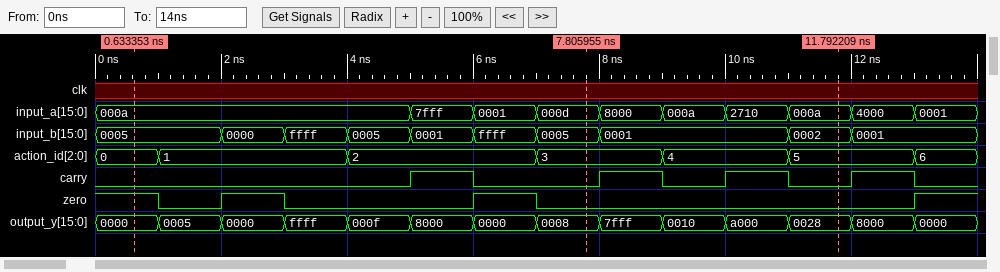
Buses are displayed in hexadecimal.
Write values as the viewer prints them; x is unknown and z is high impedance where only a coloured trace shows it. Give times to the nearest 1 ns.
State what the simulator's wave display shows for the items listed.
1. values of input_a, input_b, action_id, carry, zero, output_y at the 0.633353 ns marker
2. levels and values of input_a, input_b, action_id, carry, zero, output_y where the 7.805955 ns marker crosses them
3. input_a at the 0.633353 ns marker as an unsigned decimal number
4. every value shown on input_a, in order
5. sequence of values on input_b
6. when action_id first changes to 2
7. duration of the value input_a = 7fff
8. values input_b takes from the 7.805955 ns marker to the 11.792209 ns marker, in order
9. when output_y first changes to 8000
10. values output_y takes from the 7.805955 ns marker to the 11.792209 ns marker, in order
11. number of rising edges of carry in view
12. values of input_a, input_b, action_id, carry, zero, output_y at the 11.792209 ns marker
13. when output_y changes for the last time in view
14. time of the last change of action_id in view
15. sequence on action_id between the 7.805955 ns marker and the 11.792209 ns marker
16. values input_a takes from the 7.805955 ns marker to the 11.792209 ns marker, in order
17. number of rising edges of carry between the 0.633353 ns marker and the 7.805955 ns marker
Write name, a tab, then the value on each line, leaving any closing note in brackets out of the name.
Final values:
values of input_a, input_b, action_id, carry, zero, output_y at the 0.633353 ns marker	input_a=000a, input_b=0005, action_id=0, carry=0, zero=1, output_y=0000
levels and values of input_a, input_b, action_id, carry, zero, output_y where the 7.805955 ns marker crosses them	input_a=000d, input_b=0005, action_id=3, carry=0, zero=0, output_y=0008
input_a at the 0.633353 ns marker as an unsigned decimal number	10
every value shown on input_a, in order	000a, 7fff, 0001, 000d, 8000, 000a, 2710, 000a, 4000, 0001
sequence of values on input_b	0005, 0000, ffff, 0005, 0001, ffff, 0005, 0001, 0002, 0001
when action_id first changes to 2	4 ns
duration of the value input_a = 7fff	1 ns
values input_b takes from the 7.805955 ns marker to the 11.792209 ns marker, in order	0005, 0001, 0002
when output_y first changes to 8000	5 ns
values output_y takes from the 7.805955 ns marker to the 11.792209 ns marker, in order	0008, 7fff, 0010, a000, 0028
number of rising edges of carry in view	4
values of input_a, input_b, action_id, carry, zero, output_y at the 11.792209 ns marker	input_a=000a, input_b=0002, action_id=5, carry=0, zero=0, output_y=0028
when output_y changes for the last time in view	13 ns
time of the last change of action_id in view	13 ns
sequence on action_id between the 7.805955 ns marker and the 11.792209 ns marker	3, 4, 5
values input_a takes from the 7.805955 ns marker to the 11.792209 ns marker, in order	000d, 8000, 000a, 2710, 000a
number of rising edges of carry between the 0.633353 ns marker and the 7.805955 ns marker	1
